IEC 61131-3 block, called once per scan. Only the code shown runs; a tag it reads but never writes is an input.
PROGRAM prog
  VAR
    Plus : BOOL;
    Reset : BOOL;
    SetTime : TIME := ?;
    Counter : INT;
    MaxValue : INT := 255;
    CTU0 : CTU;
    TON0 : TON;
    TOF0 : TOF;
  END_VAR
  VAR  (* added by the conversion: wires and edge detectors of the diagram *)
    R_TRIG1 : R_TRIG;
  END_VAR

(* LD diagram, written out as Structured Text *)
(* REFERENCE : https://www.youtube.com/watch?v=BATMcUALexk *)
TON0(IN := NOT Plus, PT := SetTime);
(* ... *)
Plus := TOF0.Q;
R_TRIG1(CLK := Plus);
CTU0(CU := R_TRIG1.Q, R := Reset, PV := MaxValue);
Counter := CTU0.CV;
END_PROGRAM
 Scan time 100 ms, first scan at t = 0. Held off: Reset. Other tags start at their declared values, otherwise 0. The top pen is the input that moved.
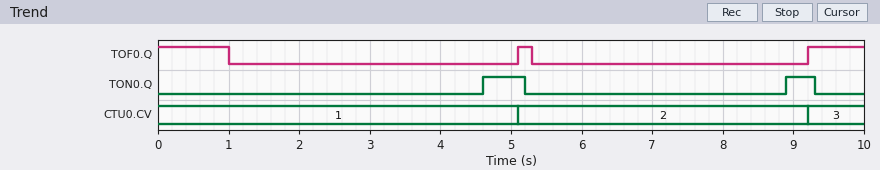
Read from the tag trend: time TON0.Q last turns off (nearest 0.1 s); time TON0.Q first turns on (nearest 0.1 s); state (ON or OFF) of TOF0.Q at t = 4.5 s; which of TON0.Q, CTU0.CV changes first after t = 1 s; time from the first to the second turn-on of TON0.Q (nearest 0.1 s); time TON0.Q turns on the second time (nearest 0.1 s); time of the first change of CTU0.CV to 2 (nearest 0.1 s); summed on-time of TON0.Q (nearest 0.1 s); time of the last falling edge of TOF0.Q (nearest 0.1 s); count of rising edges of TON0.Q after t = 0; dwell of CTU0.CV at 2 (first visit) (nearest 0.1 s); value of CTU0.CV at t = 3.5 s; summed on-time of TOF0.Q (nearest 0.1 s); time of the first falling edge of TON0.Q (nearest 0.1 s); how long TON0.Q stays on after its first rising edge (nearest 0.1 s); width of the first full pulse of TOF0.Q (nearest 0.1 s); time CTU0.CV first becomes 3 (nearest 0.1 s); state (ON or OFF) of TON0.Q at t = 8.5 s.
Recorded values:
9.3 s
4.6 s
OFF
TON0.Q
4.3 s
8.9 s
5.1 s
1.0 s
5.3 s
2
4.1 s
1
2.0 s
5.2 s
0.6 s
0.2 s
9.2 s
OFF
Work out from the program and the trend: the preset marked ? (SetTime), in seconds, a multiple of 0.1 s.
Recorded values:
3.5 s
